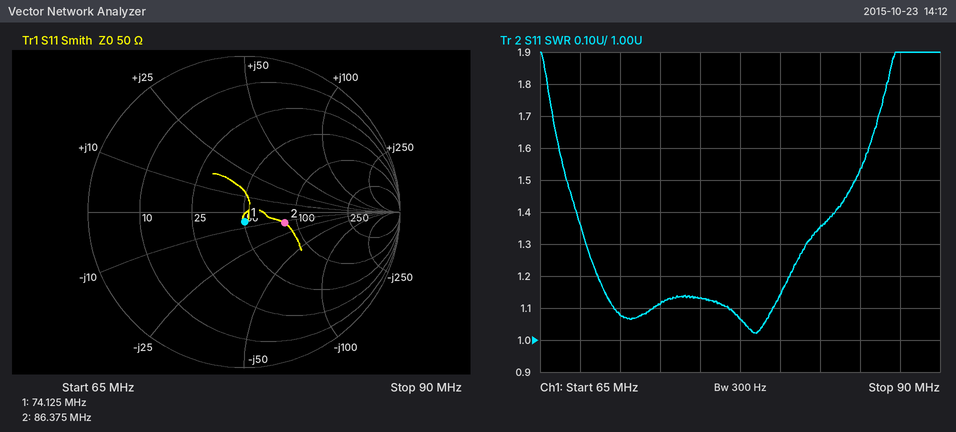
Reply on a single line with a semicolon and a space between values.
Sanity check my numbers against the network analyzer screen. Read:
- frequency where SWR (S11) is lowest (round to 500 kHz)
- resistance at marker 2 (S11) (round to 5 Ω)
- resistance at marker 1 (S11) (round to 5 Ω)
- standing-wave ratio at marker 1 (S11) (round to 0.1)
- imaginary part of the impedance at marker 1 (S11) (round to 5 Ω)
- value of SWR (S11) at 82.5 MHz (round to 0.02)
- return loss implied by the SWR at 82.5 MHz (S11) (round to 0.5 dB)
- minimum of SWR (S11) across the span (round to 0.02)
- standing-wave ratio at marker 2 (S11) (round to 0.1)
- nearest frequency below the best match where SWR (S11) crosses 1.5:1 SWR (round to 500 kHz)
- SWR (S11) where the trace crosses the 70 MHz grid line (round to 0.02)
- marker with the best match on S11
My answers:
78.5 MHz; 85 Ω; 50 Ω; 1.1; -5 Ω; 1.36; 16.5 dB; 1.02; 1.7; 66.5 MHz; 1.08; marker 1
